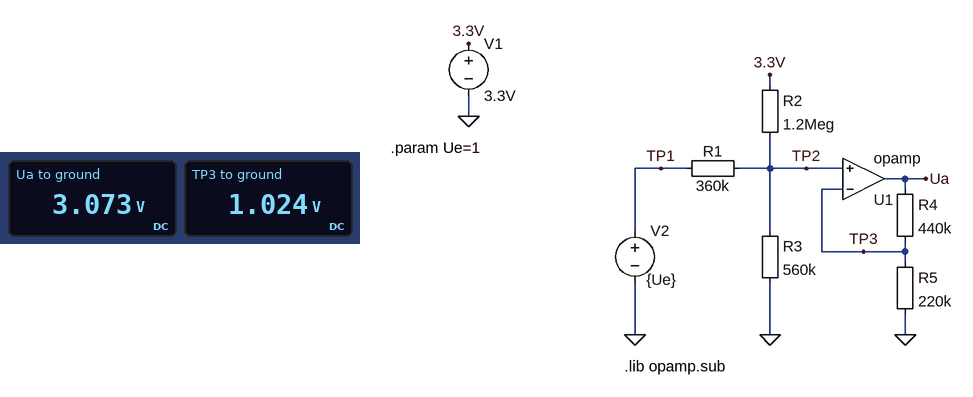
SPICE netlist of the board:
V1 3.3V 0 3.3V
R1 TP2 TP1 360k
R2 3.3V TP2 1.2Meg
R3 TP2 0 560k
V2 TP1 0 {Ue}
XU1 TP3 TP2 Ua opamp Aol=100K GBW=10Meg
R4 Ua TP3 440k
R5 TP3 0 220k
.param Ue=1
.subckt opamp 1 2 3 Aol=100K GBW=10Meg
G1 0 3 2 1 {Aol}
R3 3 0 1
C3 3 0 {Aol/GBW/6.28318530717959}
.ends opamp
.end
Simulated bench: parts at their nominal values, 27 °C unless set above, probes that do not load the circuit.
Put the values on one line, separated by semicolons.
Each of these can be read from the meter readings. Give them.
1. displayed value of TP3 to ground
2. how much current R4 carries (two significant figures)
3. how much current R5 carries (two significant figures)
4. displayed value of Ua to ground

1.024 V; 4.7 µA; 4.7 µA; 3.073 V
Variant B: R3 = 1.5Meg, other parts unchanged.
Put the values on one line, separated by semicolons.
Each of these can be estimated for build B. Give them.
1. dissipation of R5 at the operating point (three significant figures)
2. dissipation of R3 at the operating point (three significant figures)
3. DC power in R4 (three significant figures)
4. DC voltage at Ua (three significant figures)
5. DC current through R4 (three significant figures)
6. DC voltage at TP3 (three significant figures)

7.59 µW; 1.11 µW; 15.2 µW; 3.88 V; 5.87 µA; 1.29 V
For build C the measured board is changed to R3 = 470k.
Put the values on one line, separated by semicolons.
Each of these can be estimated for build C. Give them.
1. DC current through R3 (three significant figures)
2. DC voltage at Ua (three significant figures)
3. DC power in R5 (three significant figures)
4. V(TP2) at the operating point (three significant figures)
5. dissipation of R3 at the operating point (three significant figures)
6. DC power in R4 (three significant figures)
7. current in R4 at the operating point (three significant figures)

2.05 µA; 2.89 V; 4.22 µW; 963 mV; 1.97 µW; 8.43 µW; 4.38 µA
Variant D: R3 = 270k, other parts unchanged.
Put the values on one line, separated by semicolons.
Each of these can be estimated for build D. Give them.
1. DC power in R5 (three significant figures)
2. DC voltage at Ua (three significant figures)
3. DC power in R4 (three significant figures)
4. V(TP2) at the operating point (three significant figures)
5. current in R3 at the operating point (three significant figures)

2.60 µW; 2.27 V; 5.19 µW; 756 mV; 2.80 µA
